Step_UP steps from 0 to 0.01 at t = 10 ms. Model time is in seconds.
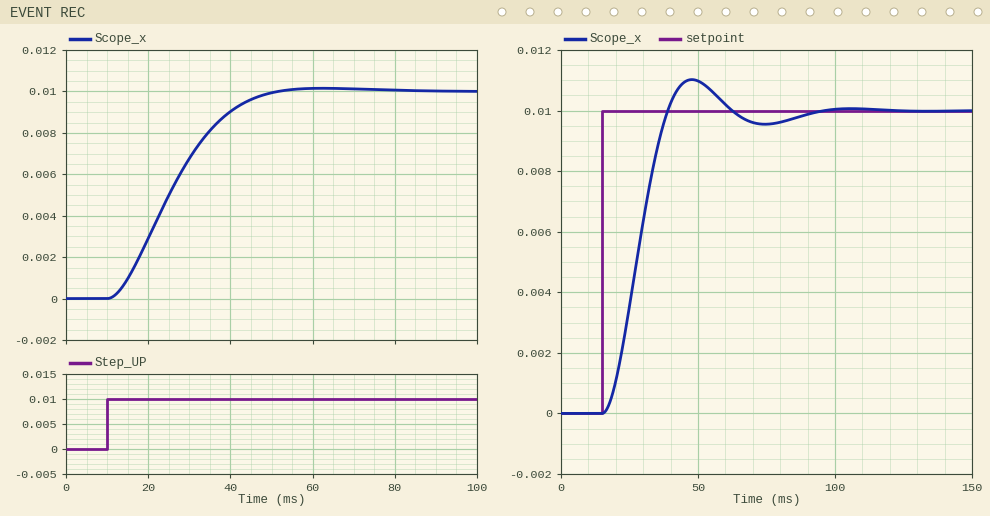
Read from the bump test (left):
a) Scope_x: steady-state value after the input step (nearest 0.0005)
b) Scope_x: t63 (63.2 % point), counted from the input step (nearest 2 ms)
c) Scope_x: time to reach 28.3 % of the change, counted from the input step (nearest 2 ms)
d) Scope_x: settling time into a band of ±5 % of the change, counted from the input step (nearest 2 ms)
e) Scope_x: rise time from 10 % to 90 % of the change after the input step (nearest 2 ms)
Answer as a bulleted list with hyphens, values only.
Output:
- 0.0100
- 18 ms
- 10 ms
- 34 ms
- 24 ms
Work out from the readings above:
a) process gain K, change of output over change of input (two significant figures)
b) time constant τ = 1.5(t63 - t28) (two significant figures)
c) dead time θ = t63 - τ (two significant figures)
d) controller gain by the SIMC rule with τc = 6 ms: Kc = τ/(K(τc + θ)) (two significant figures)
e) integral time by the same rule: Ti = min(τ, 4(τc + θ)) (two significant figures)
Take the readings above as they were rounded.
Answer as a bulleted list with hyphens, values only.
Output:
- 1.0
- 12 ms
- 6.0 ms
- 1.0
- 12 ms
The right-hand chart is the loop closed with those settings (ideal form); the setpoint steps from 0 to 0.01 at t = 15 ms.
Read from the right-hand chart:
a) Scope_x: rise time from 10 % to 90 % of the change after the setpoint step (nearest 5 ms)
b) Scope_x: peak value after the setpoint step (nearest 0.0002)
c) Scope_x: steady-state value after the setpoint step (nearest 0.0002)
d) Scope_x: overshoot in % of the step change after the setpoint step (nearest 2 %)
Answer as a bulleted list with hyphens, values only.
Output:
- 15 ms
- 0.0110
- 0.0100
- 10 %
